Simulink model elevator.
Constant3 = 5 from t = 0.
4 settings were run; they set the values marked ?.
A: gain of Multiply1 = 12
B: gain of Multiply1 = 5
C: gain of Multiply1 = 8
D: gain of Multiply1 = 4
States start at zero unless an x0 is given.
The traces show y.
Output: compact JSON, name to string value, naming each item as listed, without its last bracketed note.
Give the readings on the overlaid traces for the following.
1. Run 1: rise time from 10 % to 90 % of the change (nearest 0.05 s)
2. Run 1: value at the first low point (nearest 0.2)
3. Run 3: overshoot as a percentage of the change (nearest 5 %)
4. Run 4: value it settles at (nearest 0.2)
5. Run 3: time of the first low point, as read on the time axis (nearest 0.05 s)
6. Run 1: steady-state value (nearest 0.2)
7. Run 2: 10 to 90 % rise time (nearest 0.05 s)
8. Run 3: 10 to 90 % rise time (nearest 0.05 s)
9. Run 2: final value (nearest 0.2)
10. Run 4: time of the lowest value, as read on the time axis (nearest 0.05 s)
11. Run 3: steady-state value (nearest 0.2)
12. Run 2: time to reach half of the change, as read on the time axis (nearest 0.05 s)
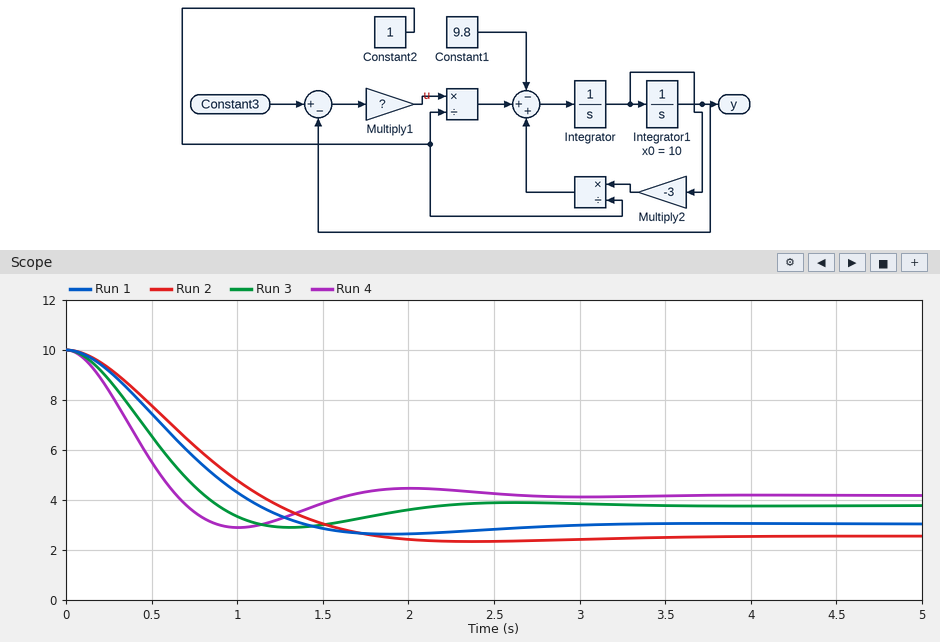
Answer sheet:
{"Run 1: rise time from 10 % to 90 % of the change": "0.90 s", "Run 1: value at the first low point": "2.6", "Run 3: overshoot as a percentage of the change": "15 %", "Run 4: value it settles at": "4.2", "Run 3: time of the first low point, as read on the time axis": "1.30 s", "Run 1: steady-state value": "3.0", "Run 2: 10 to 90 % rise time": "1.15 s", "Run 3: 10 to 90 % rise time": "0.60 s", "Run 2: final value": "2.6", "Run 4: time of the lowest value, as read on the time axis": "1.00 s", "Run 3: steady-state value": "3.8", "Run 2: time to reach half of the change, as read on the time axis": "0.75 s"}
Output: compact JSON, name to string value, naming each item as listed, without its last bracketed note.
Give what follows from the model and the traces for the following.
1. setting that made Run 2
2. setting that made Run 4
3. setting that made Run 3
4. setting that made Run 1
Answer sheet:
{"setting that made Run 2": "D", "setting that made Run 4": "A", "setting that made Run 3": "C", "setting that made Run 1": "B"}
